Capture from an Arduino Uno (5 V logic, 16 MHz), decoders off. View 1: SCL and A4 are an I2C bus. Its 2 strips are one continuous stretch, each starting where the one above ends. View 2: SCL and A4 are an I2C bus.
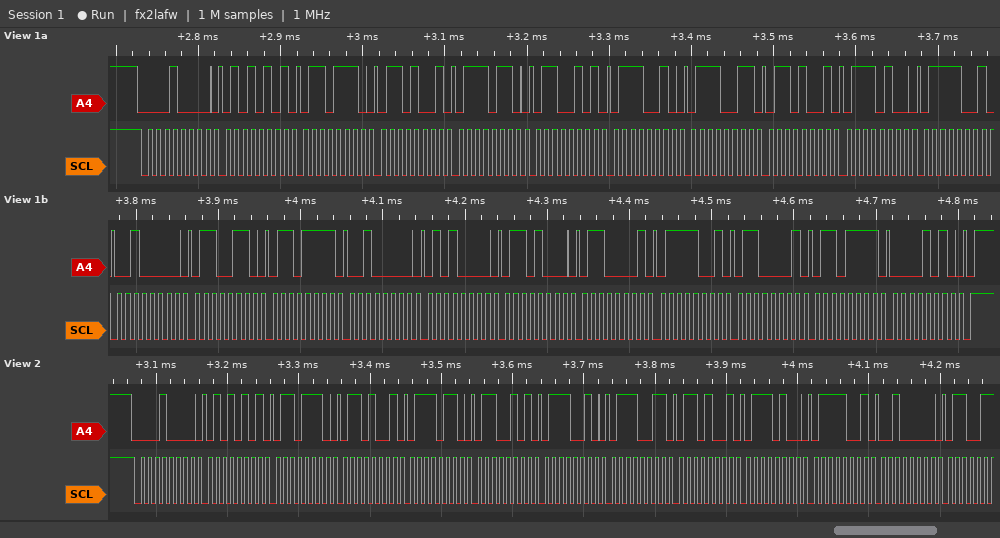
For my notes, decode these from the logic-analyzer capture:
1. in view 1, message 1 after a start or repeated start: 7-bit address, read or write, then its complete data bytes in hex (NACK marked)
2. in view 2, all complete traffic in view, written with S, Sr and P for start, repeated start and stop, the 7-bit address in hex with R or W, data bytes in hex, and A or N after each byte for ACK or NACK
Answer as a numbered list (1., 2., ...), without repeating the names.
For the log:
1. 0x08 write: 55 6E 69 76 65 72 73 69 74 79 20 66 6F 20 50 68 61 79 61 6F 0A
2. S 08W A 55 A 6E A 69 A 76 A 65 A 72 A 73 A 69 A 74 A 79 A 20 A
